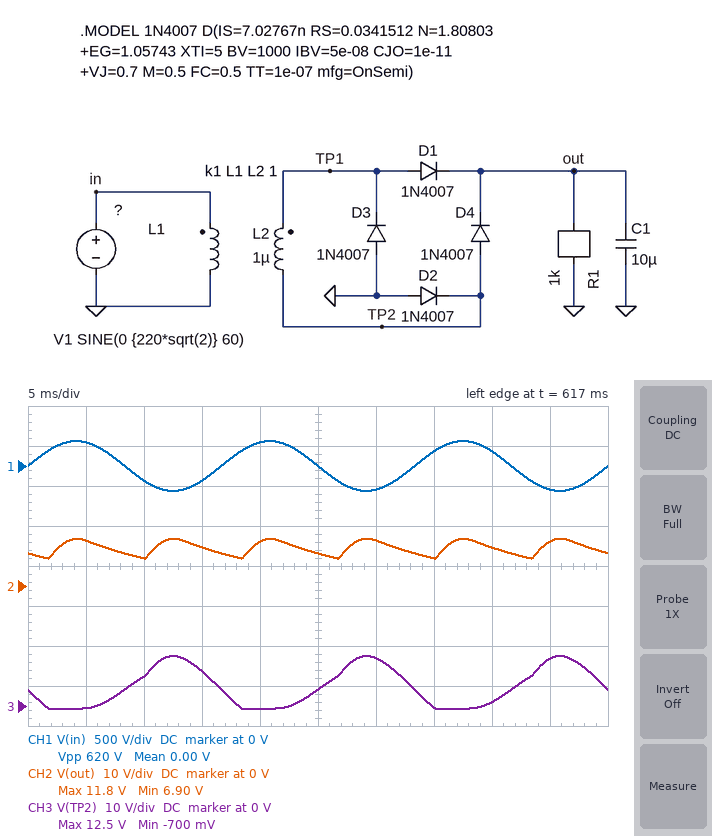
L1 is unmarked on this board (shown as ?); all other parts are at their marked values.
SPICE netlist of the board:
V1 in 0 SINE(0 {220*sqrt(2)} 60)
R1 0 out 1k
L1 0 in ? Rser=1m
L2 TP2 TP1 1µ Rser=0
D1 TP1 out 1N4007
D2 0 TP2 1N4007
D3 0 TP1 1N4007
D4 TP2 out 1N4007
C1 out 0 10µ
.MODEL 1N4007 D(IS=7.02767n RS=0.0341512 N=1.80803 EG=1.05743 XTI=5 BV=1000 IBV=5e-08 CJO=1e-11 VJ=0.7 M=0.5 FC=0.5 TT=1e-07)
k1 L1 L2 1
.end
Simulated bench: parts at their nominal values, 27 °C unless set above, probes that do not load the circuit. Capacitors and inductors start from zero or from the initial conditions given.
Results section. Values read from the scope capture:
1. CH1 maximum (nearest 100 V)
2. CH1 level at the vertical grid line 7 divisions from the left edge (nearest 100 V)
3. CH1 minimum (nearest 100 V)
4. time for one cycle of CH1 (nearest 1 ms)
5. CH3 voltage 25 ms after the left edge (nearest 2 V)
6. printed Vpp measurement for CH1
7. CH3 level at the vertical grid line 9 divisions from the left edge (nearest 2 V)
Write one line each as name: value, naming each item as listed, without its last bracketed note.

CH1 maximum: 300 V
CH1 level at the vertical grid line 7 divisions from the left edge: 200 V
CH1 minimum: -300 V
time for one cycle of CH1: 17 ms
CH3 voltage 25 ms after the left edge: 4 V
printed Vpp measurement for CH1: 620 V
CH3 level at the vertical grid line 9 divisions from the left edge: 12 V
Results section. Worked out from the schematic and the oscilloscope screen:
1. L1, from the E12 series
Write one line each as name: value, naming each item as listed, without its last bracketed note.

L1, from the E12 series: 560 µH
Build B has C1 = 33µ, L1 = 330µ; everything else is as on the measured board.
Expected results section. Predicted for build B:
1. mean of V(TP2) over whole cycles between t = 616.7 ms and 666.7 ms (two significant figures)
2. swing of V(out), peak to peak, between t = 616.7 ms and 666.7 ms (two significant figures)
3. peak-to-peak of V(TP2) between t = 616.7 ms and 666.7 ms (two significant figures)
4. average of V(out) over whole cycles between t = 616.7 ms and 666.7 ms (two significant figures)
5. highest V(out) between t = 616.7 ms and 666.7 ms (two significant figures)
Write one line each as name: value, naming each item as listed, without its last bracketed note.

mean of V(TP2) over whole cycles between t = 616.7 ms and 666.7 ms: 7.2 V
swing of V(out), peak to peak, between t = 616.7 ms and 666.7 ms: 2.8 V
peak-to-peak of V(TP2) between t = 616.7 ms and 666.7 ms: 17 V
average of V(out) over whole cycles between t = 616.7 ms and 666.7 ms: 14 V
highest V(out) between t = 616.7 ms and 666.7 ms: 16 V
